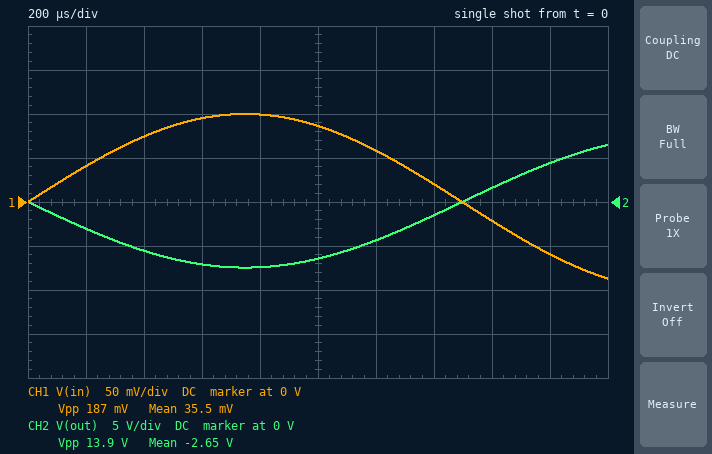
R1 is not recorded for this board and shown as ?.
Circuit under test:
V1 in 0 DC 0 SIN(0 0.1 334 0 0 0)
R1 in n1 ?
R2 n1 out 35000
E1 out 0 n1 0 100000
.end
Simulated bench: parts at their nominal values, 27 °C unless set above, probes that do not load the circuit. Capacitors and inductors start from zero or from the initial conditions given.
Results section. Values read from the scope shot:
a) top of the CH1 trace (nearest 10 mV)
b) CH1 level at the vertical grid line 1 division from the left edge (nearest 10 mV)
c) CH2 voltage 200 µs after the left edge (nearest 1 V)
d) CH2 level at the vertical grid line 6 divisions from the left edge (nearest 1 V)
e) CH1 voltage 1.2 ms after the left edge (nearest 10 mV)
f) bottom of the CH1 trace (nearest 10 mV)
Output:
100 mV
40 mV
-3 V
-4 V
60 mV
-90 mV
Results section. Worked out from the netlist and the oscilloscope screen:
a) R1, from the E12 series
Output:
470 Ω
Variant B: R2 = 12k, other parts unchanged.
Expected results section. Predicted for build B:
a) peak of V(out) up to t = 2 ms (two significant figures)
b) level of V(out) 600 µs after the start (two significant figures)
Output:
2.2 V
-2.4 V
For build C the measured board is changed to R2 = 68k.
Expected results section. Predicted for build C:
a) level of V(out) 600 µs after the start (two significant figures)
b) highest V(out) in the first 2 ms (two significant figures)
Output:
-14 V
13 V
